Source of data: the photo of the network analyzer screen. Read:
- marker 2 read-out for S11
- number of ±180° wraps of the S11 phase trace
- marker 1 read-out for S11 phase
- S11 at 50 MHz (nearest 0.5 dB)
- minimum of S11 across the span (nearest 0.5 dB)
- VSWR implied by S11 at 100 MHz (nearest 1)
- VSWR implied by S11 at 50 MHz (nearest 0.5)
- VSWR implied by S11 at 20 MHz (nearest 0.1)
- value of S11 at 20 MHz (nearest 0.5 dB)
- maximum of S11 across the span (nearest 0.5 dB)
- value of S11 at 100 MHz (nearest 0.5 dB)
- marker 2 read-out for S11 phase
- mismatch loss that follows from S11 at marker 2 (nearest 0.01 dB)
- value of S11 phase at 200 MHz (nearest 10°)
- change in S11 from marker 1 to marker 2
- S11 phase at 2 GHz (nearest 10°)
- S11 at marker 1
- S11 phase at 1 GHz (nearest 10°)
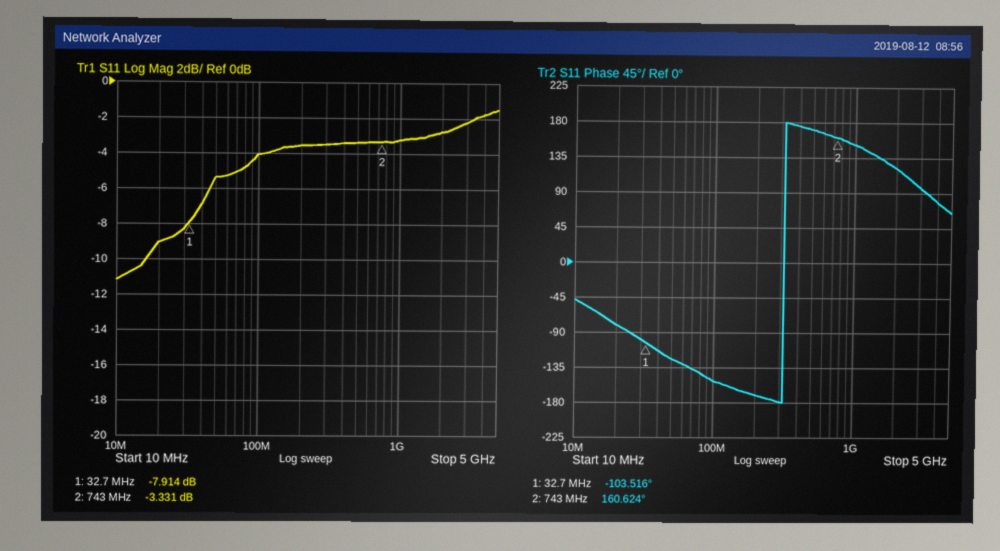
-3.331 dB
1
-103.516°
-5.5 dB
-11.0 dB
4
3.5
2.1
-9.0 dB
-1.5 dB
-4.0 dB
160.624°
2.71 dB
-170°
4.583 dB
120°
-7.914 dB
150°
